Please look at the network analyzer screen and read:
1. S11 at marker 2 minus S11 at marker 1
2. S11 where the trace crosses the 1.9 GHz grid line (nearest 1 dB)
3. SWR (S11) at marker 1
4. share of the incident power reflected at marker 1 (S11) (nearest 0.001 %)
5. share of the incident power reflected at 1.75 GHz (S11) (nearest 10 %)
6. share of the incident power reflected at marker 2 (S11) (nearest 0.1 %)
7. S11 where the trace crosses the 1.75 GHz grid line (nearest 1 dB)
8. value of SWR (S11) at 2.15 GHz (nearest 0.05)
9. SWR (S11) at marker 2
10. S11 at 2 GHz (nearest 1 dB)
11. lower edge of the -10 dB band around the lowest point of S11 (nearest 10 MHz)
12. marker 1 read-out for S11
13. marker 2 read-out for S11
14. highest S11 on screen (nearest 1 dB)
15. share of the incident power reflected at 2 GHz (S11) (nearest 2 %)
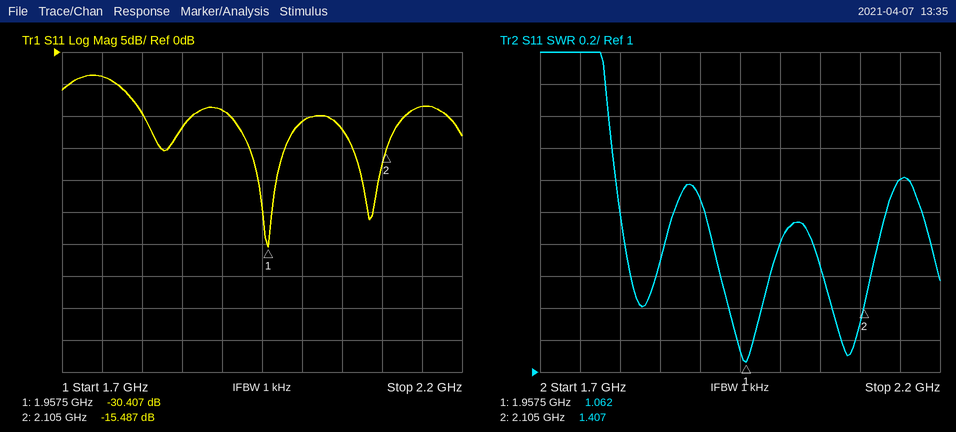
14.920 dB
-9 dB
1.062
0.091 %
40 %
2.8 %
-4 dB
2.20
1.407
-11 dB
1.91 GHz
-30.407 dB
-15.487 dB
-4 dB
8 %
